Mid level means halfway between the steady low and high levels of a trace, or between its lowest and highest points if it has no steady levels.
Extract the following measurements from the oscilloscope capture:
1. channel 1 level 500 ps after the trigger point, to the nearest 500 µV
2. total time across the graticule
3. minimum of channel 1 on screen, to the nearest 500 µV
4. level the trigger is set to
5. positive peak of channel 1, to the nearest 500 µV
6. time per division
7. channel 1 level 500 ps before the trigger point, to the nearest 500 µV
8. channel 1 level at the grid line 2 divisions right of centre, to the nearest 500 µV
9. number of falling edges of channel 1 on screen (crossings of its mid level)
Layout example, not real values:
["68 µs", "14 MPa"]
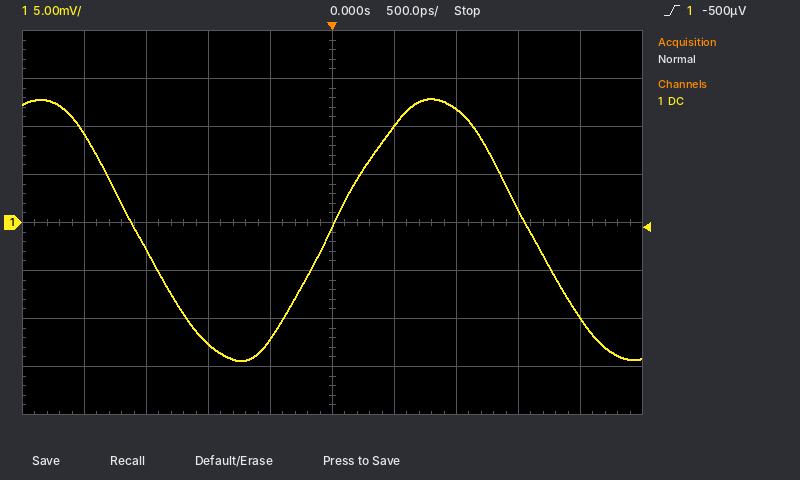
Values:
["10.0 mV", "5 ns", "-14.5 mV", "-500 µV", "13.0 mV", "500 ps", "-12.0 mV", "12.0 mV", "2"]
